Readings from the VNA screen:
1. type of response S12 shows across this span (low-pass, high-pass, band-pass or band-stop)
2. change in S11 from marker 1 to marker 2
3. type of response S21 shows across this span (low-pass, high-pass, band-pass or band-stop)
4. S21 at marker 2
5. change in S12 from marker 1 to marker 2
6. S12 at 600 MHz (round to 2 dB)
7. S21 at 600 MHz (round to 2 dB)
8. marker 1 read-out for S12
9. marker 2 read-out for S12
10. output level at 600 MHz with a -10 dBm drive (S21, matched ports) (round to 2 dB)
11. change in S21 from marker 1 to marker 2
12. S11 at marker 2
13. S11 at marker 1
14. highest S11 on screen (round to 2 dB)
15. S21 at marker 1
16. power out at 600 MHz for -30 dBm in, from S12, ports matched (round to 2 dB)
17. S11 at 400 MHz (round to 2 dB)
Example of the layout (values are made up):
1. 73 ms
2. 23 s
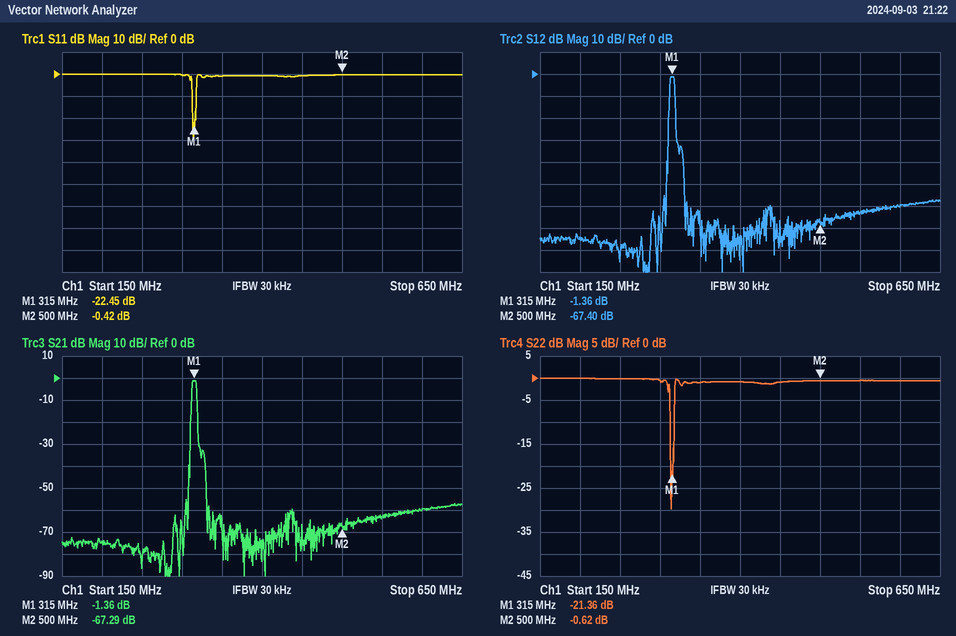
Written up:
1. band-pass
2. 22.03 dB
3. band-pass
4. -67.29 dB
5. -66.04 dB
6. -60 dB
7. -60 dB
8. -1.36 dB
9. -67.40 dB
10. -70 dBm
11. -65.93 dB
12. -0.42 dB
13. -22.45 dB
14. 0 dB
15. -1.36 dB
16. -90 dBm
17. 0 dB
